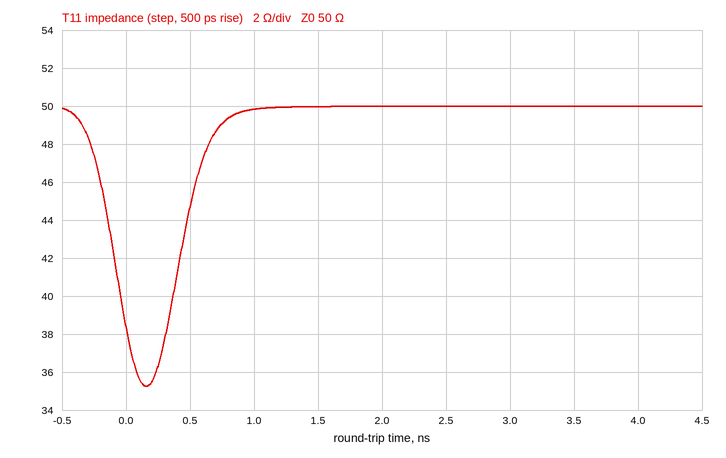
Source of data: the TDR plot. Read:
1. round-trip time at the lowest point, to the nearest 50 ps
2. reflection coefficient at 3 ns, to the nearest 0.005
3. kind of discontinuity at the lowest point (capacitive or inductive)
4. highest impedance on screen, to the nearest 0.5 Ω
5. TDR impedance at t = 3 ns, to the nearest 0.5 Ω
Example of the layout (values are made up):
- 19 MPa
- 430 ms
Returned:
- 150 ps
- 0.000
- capacitive
- 50.0 Ω
- 50.0 Ω
